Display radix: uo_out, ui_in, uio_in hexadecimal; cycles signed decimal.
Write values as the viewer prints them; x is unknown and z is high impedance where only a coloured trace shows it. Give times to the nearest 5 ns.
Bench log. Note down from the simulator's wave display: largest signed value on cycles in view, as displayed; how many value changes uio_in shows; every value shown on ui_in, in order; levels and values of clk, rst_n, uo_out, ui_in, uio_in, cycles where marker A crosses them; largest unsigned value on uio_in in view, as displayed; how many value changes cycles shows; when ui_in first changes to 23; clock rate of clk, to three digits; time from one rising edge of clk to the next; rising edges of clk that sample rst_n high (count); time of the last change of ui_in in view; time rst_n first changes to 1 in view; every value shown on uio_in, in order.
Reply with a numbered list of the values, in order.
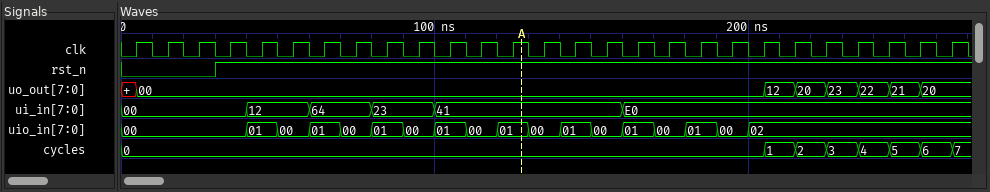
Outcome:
1. 7
2. 17
3. 00, 12, 64, 23, 41, E0
4. clk=1, rst_n=1, uo_out=00, ui_in=41, uio_in=01, cycles=0
5. 02
6. 7
7. 80 ns
8. 100 MHz
9. 10 ns
10. 24
11. 160 ns
12. 30 ns
13. 00, 01, 00, 01, 00, 01, 00, 01, 00, 01, 00, 01, 00, 01, 00, 01, 00, 02
